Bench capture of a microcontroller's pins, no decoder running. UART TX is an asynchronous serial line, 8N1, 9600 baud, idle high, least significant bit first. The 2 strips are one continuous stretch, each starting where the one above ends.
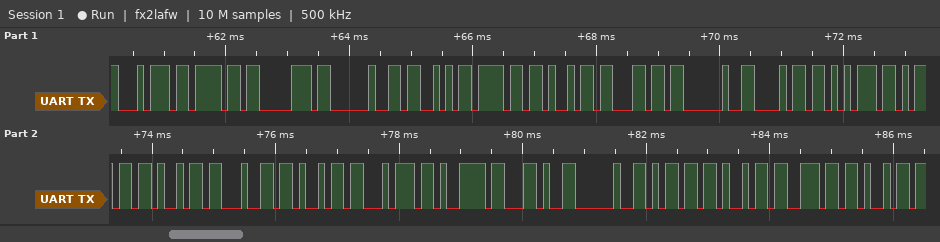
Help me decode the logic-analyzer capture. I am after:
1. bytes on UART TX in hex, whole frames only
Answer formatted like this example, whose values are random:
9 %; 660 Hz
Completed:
74 6F 70 20 53 6F 69 6C 20 68 75 6D 69 64 69 74 79 2C 20 6D 69 6E 69
